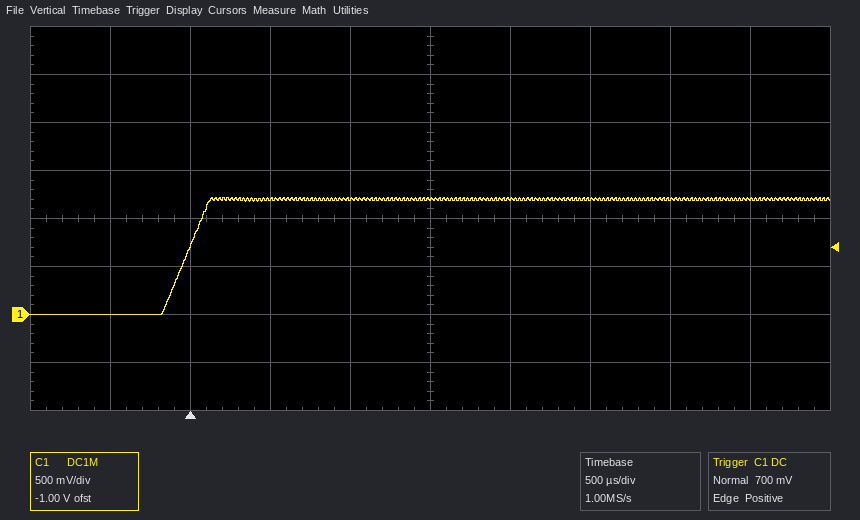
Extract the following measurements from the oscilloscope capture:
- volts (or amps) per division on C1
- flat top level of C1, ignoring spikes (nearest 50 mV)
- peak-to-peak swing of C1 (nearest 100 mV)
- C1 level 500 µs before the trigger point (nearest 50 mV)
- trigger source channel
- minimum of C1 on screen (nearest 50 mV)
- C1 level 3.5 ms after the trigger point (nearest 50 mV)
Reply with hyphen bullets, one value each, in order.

- 500 mV
- 1.20 V
- 1.20 V
- 0 mV
- C1
- 0 mV
- 1.20 V
